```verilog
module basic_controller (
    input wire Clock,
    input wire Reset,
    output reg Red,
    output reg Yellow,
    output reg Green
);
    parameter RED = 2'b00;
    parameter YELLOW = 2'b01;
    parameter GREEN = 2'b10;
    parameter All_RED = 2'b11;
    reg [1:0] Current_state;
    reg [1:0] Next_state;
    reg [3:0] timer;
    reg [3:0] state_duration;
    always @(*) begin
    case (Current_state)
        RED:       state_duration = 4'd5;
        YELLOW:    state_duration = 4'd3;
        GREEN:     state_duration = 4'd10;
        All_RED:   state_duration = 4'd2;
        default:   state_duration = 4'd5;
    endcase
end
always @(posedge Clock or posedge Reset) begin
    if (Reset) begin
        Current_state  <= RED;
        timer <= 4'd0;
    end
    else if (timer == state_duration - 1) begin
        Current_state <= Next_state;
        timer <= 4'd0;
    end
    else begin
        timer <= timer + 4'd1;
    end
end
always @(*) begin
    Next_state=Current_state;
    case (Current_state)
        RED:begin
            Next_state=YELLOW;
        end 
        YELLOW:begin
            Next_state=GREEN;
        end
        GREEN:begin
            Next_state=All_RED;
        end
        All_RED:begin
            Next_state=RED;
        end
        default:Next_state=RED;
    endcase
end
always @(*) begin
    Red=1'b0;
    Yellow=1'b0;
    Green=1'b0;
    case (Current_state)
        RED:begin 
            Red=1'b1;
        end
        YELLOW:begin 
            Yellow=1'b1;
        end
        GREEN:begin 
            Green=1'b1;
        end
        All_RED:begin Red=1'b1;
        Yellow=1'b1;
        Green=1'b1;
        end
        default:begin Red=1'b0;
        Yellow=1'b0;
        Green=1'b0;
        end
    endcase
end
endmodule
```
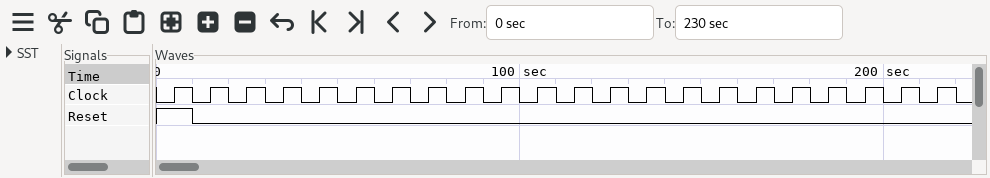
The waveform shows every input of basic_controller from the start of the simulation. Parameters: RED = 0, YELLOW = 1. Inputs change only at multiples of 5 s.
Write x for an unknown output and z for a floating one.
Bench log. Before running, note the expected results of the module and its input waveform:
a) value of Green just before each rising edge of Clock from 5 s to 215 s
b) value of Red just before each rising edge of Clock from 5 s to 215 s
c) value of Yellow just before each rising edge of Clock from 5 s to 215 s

0 0 0 0 0 0 0 0 0 1 1 1 1 1 1 1 1 1 1 1 1 0
1 1 1 1 1 1 0 0 0 0 0 0 0 0 0 0 0 0 0 1 1 1
0 0 0 0 0 0 1 1 1 0 0 0 0 0 0 0 0 0 0 1 1 0
